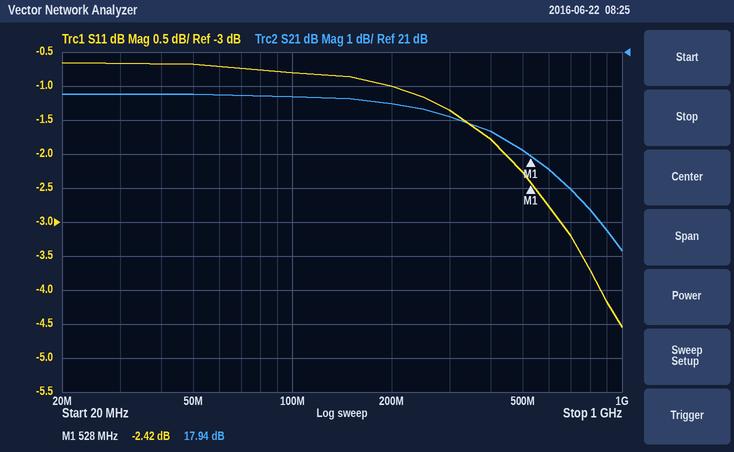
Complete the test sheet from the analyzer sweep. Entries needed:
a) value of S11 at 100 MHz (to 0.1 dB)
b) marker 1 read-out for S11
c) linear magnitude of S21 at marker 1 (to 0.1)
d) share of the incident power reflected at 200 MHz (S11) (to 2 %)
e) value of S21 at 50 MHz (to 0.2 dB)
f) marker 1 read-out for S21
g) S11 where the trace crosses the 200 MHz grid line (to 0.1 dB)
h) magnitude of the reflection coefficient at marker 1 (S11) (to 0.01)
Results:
-0.8 dB
-2.42 dB
7.9
80 %
19.8 dB
17.94 dB
-1.0 dB
0.76
